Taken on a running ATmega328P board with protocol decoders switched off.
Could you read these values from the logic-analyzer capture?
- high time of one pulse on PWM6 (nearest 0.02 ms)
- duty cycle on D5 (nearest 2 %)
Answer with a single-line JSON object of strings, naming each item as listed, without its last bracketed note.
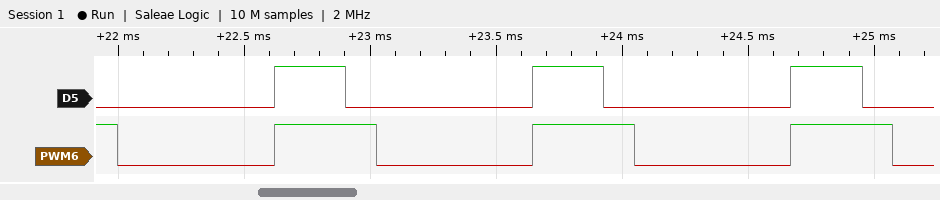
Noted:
{"high time of one pulse on PWM6": "0.40 ms", "duty cycle on D5": "28 %"}
